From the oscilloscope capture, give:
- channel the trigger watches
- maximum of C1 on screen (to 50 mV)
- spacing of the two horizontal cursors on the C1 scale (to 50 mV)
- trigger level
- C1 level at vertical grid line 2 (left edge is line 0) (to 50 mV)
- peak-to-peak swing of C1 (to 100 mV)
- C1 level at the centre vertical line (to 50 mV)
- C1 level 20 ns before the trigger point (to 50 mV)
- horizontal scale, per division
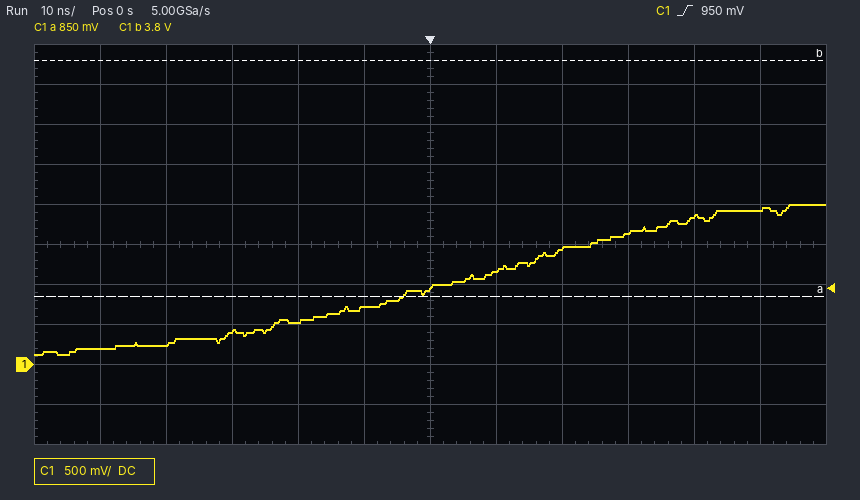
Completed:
C1
2.00 V
2.95 V
950 mV
250 mV
1.90 V
950 mV
550 mV
10 ns
